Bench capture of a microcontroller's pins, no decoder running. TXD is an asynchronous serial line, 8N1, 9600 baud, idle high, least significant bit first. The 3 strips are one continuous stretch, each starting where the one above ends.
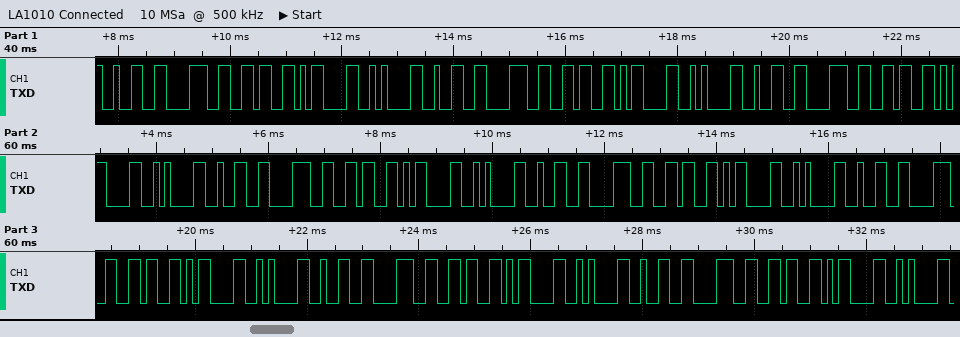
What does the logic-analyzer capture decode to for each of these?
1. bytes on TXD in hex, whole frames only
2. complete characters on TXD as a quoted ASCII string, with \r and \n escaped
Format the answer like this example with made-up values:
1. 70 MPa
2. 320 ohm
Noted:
1. 32 38 36 0D 0A 32 38 36 0D 0A 32 38 36 0D 0A 32 38 36 0D 0A 32 38 36 0D 0A 32 38 36 0D 0A 32 38 36 0D 0A 32 38 36 0D 0A
2. "286\r\n286\r\n286\r\n286\r\n286\r\n286\r\n286\r\n286\r\n"
